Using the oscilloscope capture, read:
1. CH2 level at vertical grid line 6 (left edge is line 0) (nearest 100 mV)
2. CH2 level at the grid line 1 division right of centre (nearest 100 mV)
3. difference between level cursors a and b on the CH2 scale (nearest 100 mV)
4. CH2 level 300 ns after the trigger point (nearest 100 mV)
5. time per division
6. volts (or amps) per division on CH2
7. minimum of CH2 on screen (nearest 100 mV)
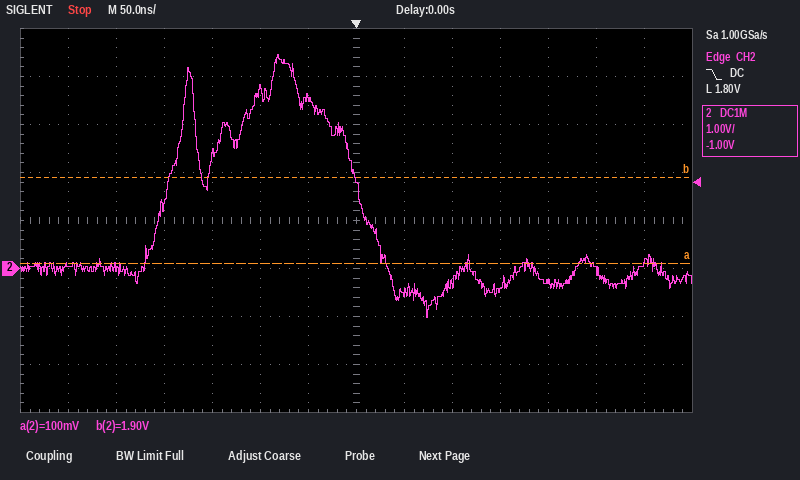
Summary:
3.6 V
-500 mV
1.8 V
100 mV
50 ns
1 V
-1.0 V
